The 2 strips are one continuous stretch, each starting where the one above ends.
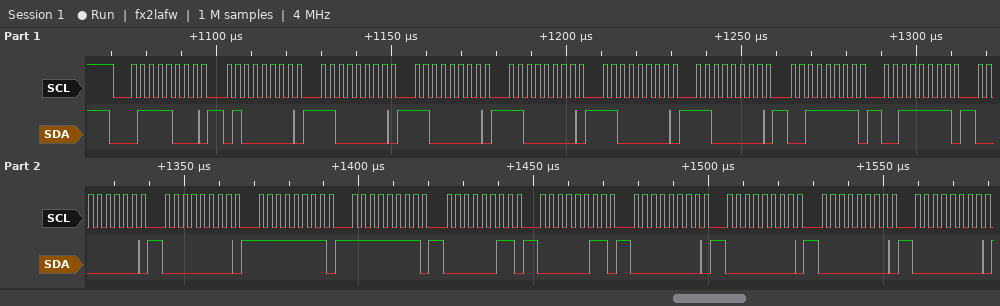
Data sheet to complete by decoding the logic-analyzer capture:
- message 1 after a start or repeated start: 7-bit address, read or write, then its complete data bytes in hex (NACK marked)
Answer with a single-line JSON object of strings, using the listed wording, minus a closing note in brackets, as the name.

{"message 1 after a start or repeated start: 7-bit address, read or write, then its complete data bytes in hex": "0x3C write: 40 C0 C0 C0 C0 C0 3F 3F 00 00 FF FF 03 03 00 00 00 00"}
